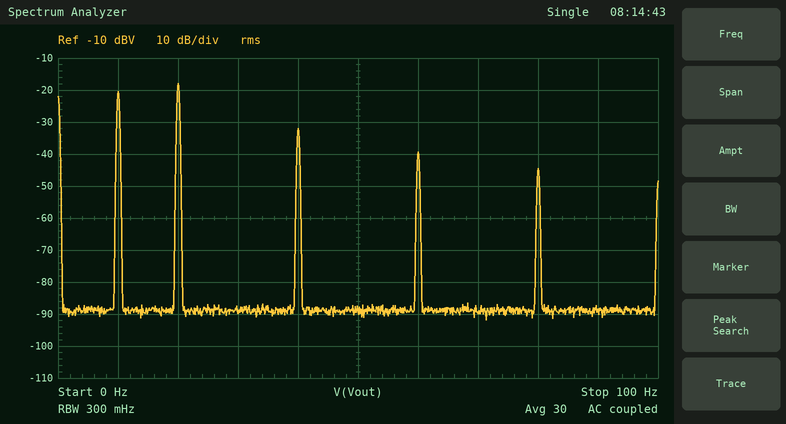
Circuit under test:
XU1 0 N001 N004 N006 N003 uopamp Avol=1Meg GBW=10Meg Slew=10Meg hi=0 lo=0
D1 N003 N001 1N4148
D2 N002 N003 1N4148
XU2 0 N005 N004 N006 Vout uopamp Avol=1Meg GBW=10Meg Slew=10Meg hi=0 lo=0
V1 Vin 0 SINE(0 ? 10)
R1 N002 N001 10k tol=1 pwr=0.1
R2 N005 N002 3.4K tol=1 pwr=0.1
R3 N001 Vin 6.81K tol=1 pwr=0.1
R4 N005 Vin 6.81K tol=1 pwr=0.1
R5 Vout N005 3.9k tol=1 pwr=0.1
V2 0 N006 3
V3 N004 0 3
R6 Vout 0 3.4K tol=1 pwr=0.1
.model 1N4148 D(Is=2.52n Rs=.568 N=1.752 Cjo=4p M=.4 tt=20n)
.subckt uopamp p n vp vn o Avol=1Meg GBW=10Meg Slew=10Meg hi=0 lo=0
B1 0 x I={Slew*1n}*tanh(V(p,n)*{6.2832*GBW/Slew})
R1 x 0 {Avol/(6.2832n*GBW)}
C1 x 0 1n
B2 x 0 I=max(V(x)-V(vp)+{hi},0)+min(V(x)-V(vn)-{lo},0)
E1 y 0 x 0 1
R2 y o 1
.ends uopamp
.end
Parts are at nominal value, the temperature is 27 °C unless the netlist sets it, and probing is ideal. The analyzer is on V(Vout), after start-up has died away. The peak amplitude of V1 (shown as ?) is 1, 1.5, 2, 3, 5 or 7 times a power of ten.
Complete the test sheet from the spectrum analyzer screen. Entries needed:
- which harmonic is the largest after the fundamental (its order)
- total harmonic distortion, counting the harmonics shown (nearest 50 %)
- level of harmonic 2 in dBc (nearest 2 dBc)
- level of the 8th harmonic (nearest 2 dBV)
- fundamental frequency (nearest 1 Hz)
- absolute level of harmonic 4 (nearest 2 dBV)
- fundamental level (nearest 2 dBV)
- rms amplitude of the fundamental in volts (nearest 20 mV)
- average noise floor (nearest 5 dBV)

2
150 %
2 dBc
-44 dBV
10 Hz
-32 dBV
-20 dBV
100 mV
-90 dBV
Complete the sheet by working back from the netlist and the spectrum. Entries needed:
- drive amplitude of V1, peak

500 mV
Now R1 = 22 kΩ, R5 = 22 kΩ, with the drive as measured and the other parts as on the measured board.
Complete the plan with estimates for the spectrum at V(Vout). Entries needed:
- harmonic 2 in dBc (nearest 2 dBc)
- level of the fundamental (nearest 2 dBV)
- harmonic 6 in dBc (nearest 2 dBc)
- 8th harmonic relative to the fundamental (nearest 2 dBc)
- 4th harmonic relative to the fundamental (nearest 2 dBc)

-4 dBc
-2 dBV
-12 dBc
-16 dBc
-10 dBc
